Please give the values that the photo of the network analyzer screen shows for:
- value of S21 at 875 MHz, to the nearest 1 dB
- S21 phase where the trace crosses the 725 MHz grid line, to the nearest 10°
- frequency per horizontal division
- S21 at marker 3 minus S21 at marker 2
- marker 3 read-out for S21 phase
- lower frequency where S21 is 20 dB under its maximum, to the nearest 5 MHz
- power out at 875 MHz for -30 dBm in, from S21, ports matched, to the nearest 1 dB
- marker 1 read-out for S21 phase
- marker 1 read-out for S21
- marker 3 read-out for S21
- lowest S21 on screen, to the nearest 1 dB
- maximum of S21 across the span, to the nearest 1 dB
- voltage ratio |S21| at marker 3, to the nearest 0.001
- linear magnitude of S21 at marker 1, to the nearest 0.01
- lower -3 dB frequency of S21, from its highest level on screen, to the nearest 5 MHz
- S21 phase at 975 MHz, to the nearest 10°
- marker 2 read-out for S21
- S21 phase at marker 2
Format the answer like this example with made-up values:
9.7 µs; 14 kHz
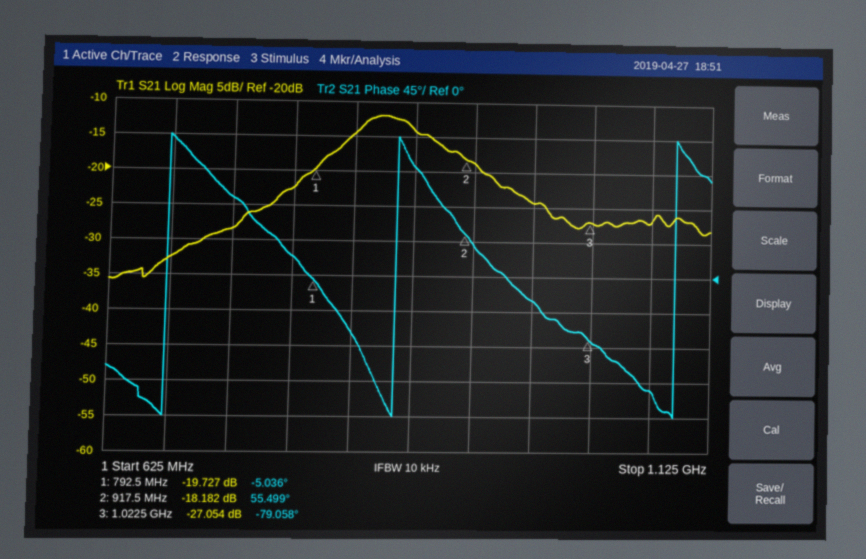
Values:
-14 dB; 100°; 50 MHz; -8.872 dB; -79.058°; 680 MHz; -44 dBm; -5.036°; -19.727 dB; -27.054 dB; -36 dB; -12 dB; 0.044; 0.10; 820 MHz; -30°; -18.182 dB; 55.499°
